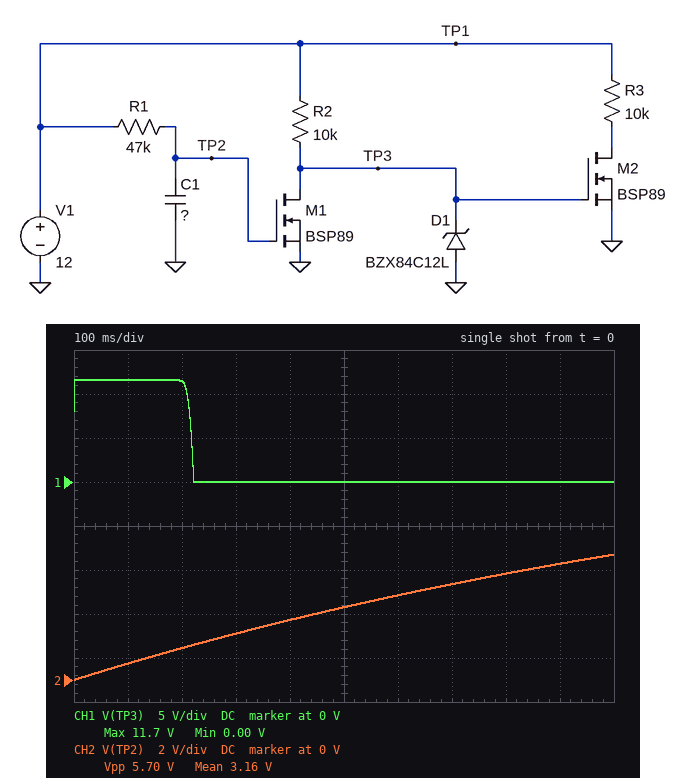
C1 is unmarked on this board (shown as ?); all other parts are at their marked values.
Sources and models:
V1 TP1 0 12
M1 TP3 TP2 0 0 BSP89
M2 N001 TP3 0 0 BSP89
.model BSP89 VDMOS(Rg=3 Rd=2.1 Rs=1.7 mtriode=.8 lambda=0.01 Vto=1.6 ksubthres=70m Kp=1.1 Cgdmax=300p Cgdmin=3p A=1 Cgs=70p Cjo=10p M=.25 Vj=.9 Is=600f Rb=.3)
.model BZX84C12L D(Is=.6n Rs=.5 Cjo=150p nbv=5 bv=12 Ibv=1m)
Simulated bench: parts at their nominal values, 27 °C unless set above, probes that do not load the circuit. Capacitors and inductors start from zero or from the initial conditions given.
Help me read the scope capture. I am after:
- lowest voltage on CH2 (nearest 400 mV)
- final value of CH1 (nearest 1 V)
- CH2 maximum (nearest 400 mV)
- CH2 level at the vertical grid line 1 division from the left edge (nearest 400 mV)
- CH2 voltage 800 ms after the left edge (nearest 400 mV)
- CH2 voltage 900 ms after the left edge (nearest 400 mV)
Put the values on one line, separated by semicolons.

0 V; 0 V; 5.6 V; 800 mV; 4.8 V; 5.2 V
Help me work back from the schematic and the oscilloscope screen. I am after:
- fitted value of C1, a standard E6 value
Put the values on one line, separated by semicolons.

33 µF
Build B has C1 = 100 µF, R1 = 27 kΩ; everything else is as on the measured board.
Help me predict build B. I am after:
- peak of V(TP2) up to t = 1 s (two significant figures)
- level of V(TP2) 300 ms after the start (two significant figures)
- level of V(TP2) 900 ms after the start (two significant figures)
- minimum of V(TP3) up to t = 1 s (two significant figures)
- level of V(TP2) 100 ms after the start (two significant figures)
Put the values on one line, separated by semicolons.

3.7 V; 1.3 V; 3.4 V; 5.2 mV; 440 mV
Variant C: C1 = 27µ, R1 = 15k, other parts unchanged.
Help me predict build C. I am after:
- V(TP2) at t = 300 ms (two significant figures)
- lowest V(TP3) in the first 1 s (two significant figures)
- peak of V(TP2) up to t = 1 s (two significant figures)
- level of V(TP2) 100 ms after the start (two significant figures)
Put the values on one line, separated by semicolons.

6.3 V; 4.7 mV; 11 V; 2.6 V
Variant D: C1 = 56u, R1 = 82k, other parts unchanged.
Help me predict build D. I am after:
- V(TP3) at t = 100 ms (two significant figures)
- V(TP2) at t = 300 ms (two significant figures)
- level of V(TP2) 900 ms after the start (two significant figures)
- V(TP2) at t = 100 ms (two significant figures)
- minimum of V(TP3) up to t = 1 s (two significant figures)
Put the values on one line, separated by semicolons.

12 V; 760 mV; 2.1 V; 260 mV; 6.4 mV
